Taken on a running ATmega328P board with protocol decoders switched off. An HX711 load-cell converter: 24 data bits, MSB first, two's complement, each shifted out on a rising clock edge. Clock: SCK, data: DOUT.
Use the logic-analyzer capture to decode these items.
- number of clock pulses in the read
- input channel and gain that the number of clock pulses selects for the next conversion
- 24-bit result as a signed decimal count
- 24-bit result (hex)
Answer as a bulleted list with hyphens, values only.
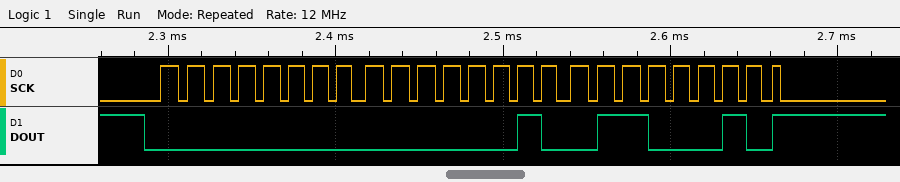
- 25
- channel A, gain 128
- 610
- 0x000262
